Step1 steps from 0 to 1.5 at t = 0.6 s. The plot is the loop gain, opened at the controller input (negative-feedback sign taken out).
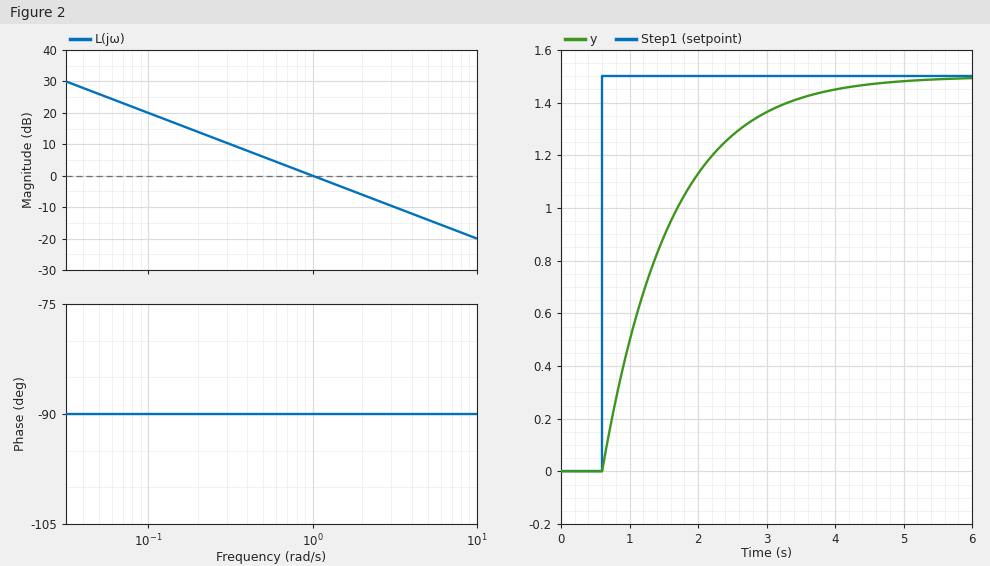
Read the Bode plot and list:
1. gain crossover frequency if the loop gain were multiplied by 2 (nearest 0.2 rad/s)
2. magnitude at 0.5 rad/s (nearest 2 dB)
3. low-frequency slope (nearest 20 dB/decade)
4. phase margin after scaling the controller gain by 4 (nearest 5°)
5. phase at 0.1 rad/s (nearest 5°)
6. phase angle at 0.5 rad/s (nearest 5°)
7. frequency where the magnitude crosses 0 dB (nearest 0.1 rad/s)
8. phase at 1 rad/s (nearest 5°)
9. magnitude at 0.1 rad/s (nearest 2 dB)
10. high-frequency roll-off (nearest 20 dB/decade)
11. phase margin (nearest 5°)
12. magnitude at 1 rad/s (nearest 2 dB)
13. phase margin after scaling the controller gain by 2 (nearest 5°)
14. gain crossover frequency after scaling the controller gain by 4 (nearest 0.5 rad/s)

2.0 rad/s
6 dB
-20 dB/decade
90°
-90°
-90°
1.0 rad/s
-90°
20 dB
-20 dB/decade
90°
0 dB
90°
4.0 rad/s
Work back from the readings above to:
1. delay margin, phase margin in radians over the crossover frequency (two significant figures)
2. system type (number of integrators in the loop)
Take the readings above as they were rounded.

1.6 s
1
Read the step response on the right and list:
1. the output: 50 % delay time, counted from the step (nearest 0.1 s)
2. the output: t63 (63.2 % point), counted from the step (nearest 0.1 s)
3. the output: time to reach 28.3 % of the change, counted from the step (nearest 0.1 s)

0.7 s
1.0 s
0.3 s
